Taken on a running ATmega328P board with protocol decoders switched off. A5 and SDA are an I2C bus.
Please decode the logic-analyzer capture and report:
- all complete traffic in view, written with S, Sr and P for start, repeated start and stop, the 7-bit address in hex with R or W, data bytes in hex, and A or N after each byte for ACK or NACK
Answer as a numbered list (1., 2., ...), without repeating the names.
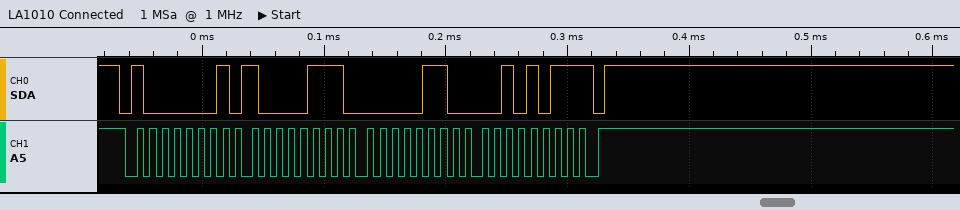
1. S 40R A 87 A 06 A 2B N P
